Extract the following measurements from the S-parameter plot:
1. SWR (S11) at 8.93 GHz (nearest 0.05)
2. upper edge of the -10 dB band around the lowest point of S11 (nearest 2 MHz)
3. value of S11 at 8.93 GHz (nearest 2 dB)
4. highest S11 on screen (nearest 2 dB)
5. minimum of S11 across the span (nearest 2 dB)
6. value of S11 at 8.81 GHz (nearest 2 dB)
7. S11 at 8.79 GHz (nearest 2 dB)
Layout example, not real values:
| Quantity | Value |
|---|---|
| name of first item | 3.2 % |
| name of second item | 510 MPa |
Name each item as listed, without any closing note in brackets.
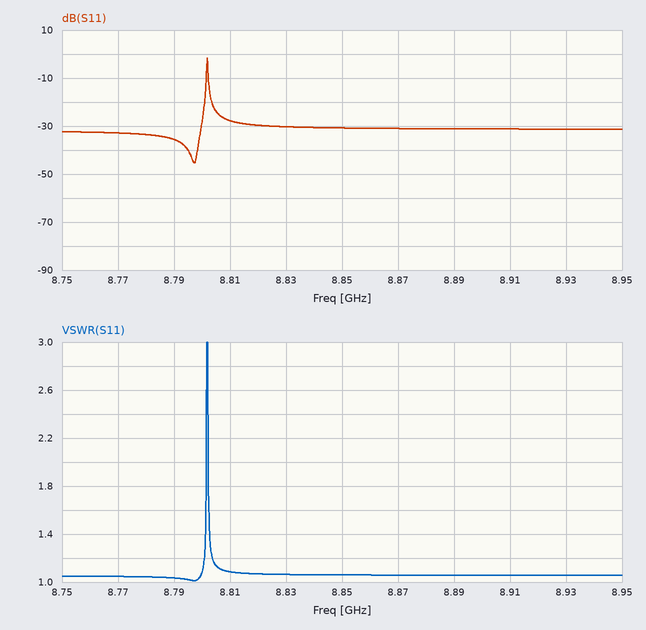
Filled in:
| Quantity | Value |
|---|---|
| SWR (S11) at 8.93 GHz | 1.05 |
| upper edge of the -10 dB band around the lowest point of S11 | 8.802 GHz |
| value of S11 at 8.93 GHz | -32 dB |
| highest S11 on screen | -2 dB |
| minimum of S11 across the span | -46 dB |
| value of S11 at 8.81 GHz | -28 dB |
| S11 at 8.79 GHz | -36 dB |
